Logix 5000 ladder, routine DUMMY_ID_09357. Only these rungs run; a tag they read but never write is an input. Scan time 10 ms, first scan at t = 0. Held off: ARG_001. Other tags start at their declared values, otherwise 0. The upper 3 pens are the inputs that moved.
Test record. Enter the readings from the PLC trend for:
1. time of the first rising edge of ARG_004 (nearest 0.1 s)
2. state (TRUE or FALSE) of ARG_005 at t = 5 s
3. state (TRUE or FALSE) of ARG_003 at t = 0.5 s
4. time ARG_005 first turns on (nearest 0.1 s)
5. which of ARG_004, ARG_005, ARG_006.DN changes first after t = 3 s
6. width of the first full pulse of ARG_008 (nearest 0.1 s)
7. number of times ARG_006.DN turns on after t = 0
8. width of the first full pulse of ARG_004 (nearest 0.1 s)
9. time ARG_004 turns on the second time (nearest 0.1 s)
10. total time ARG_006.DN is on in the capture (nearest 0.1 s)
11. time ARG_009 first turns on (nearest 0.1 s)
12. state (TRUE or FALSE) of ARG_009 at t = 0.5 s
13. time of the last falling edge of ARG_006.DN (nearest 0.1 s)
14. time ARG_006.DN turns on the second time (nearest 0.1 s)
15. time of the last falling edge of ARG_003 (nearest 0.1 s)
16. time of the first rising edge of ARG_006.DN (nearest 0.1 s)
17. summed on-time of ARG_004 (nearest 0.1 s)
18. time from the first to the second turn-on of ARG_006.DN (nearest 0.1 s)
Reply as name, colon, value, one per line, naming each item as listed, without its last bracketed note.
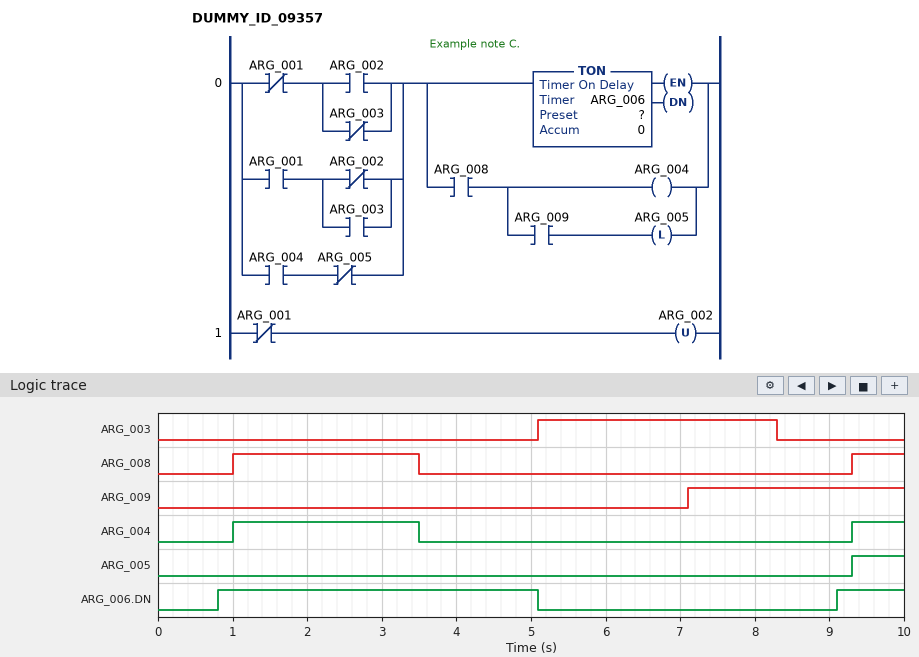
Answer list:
time of the first rising edge of ARG_004: 1.0 s
state (TRUE or FALSE) of ARG_005 at t = 5 s: FALSE
state (TRUE or FALSE) of ARG_003 at t = 0.5 s: FALSE
time ARG_005 first turns on: 9.3 s
which of ARG_004, ARG_005, ARG_006.DN changes first after t = 3 s: ARG_004
width of the first full pulse of ARG_008: 2.5 s
number of times ARG_006.DN turns on after t = 0: 2
width of the first full pulse of ARG_004: 2.5 s
time ARG_004 turns on the second time: 9.3 s
total time ARG_006.DN is on in the capture: 5.2 s
time ARG_009 first turns on: 7.1 s
state (TRUE or FALSE) of ARG_009 at t = 0.5 s: FALSE
time of the last falling edge of ARG_006.DN: 5.1 s
time ARG_006.DN turns on the second time: 9.1 s
time of the last falling edge of ARG_003: 8.3 s
time of the first rising edge of ARG_006.DN: 0.8 s
summed on-time of ARG_004: 3.2 s
time from the first to the second turn-on of ARG_006.DN: 8.3 s
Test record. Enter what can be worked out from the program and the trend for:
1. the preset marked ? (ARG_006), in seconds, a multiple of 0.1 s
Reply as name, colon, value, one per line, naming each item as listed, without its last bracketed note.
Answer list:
the preset marked ? (ARG_006), in seconds, a multiple of 0.1 s: 0.8 s
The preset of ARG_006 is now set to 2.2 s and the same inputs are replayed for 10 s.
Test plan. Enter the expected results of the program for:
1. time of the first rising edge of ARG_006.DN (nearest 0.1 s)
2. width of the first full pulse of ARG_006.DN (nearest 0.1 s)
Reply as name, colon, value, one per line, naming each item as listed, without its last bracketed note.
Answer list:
time of the first rising edge of ARG_006.DN: 2.2 s
width of the first full pulse of ARG_006.DN: 2.9 s
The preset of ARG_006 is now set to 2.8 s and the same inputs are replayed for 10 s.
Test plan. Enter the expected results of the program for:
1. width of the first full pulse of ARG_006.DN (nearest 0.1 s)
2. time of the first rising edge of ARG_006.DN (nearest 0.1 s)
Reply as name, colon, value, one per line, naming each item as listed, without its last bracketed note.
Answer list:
width of the first full pulse of ARG_006.DN: 2.3 s
time of the first rising edge of ARG_006.DN: 2.8 s
